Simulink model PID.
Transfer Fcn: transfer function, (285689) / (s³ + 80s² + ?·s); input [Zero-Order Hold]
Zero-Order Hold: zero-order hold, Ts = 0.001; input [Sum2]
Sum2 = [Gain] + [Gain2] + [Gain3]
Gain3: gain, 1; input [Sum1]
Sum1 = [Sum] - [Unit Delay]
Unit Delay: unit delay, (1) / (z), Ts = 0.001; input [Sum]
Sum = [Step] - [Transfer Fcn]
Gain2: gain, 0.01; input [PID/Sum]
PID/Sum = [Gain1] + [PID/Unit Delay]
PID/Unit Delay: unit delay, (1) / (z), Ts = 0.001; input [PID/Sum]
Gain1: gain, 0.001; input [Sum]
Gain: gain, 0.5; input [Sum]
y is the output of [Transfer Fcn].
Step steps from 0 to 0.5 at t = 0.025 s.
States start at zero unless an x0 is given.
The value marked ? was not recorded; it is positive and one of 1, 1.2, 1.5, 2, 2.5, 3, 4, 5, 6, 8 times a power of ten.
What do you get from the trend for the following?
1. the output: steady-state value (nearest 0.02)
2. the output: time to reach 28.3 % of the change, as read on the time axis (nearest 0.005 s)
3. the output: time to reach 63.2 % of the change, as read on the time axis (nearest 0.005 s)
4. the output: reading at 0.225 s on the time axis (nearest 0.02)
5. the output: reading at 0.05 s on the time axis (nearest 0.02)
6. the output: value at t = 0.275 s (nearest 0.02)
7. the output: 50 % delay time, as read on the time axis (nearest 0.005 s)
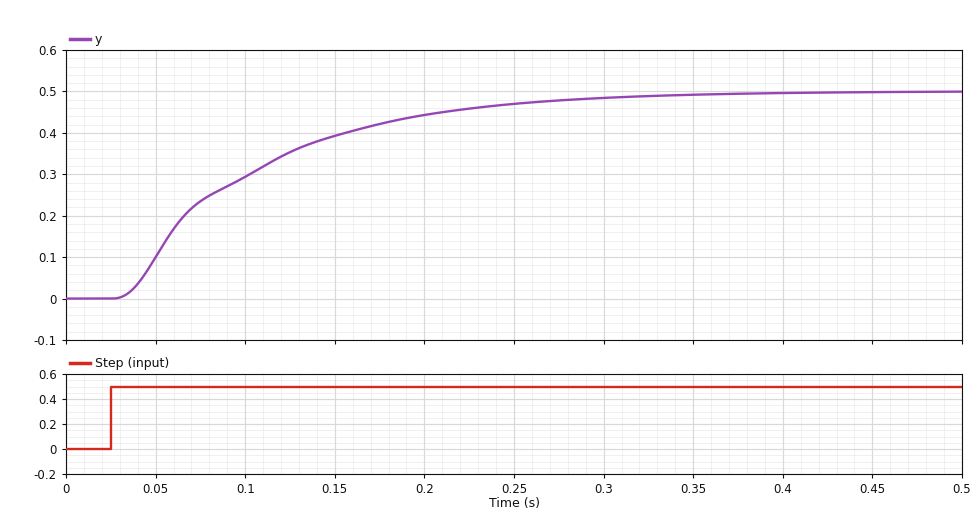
0.50
0.055 s
0.110 s
0.46
0.10
0.48
0.080 s
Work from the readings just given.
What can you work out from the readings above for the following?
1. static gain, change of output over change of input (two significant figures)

1.0
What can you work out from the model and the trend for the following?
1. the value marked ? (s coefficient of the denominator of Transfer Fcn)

12000
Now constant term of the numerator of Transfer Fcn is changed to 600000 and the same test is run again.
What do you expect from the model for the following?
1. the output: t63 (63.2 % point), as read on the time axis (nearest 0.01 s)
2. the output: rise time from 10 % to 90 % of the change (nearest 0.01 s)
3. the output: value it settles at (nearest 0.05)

0.06 s
0.08 s
0.50
